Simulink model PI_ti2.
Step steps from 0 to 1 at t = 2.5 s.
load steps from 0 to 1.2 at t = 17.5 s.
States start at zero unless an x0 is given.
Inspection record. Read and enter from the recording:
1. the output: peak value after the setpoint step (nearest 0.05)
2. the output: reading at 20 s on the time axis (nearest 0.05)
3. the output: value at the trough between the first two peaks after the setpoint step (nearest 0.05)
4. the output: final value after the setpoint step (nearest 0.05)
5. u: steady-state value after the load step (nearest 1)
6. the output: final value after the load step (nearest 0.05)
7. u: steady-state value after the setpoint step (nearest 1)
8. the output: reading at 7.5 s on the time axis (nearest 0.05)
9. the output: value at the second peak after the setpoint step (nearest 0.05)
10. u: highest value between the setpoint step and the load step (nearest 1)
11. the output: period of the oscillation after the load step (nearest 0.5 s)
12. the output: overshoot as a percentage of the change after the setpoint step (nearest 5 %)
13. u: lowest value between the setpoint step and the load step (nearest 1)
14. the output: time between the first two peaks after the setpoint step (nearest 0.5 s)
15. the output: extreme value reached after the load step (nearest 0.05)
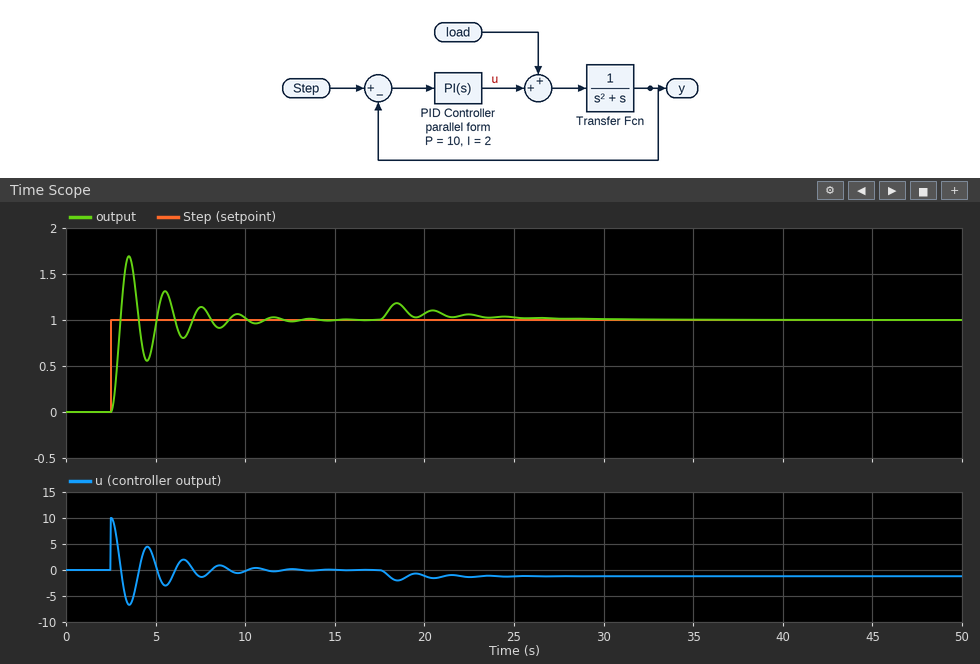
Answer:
1.70
1.05
0.55
1.00
-1
1.00
0
1.15
1.30
10
2.0 s
70 %
-7
2.0 s
1.20
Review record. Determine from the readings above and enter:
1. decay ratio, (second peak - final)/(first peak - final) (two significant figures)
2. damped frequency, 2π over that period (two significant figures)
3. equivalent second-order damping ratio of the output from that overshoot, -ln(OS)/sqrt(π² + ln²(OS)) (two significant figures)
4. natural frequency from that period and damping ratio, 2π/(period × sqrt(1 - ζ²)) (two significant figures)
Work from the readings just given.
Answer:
0.43
3.1 rad/s
0.11
3.2 rad/s
